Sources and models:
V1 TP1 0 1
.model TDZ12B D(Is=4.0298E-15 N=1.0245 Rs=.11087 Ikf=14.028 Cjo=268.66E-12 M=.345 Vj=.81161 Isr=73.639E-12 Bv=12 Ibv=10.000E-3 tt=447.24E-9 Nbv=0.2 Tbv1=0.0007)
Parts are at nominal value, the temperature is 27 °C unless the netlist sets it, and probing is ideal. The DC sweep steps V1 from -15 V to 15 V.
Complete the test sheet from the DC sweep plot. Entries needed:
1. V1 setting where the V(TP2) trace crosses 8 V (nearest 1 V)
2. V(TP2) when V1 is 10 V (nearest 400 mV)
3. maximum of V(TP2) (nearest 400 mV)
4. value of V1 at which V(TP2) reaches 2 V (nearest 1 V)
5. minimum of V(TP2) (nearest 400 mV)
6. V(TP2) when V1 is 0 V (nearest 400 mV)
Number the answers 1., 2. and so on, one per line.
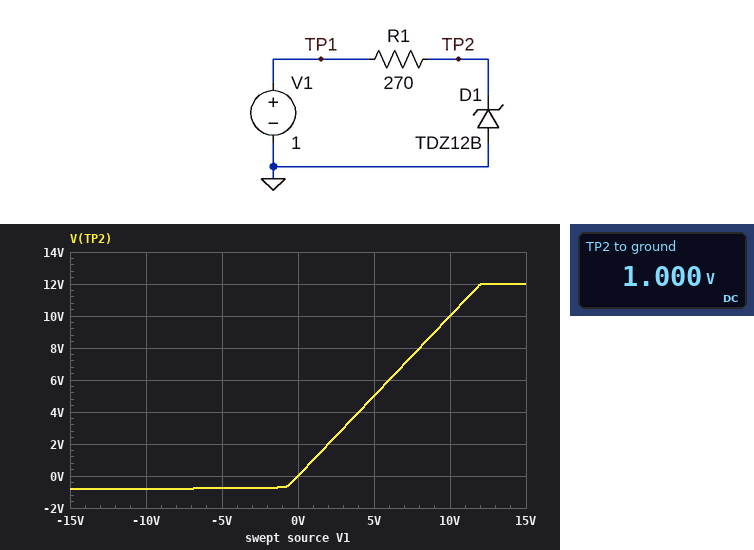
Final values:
1. 8 V
2. 10.0 V
3. 12.0 V
4. 2 V
5. -800 mV
6. 0 V
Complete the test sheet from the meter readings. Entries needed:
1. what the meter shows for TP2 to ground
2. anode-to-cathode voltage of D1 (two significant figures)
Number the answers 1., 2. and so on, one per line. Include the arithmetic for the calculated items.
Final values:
1. 1.000 V
2. 0 V - 1 V = -1.0 V
